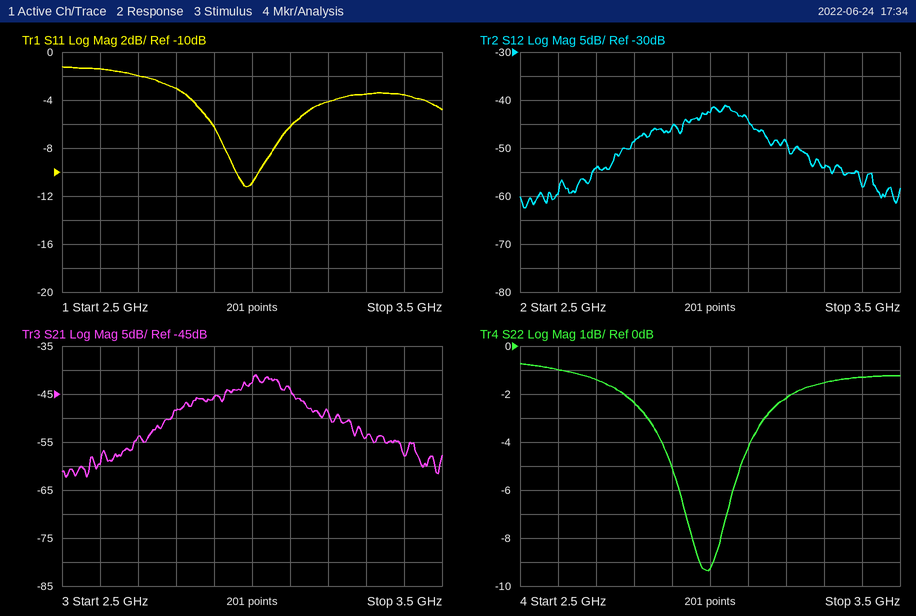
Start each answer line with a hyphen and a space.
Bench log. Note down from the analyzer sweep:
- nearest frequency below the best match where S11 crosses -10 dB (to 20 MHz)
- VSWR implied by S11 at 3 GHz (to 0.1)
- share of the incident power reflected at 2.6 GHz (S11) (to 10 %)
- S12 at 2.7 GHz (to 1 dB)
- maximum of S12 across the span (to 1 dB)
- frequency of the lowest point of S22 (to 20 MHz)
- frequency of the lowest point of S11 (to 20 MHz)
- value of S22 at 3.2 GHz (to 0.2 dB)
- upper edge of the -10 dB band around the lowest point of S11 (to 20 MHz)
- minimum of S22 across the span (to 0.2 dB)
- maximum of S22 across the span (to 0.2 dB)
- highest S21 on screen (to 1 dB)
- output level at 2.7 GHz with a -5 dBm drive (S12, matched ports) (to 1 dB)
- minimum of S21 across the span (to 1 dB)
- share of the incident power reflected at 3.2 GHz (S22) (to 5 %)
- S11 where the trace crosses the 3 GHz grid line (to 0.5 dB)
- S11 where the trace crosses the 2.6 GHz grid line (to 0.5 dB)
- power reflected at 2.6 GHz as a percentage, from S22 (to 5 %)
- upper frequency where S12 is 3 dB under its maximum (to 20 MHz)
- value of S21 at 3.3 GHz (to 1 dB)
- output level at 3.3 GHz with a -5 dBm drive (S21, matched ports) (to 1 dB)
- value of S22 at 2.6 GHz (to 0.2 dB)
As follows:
- 2.96 GHz
- 1.8
- 70 %
- -54 dB
- -41 dB
- 3.00 GHz
- 2.98 GHz
- -2.2 dB
- 3.02 GHz
- -9.4 dB
- -0.8 dB
- -41 dB
- -59 dBm
- -62 dB
- 60 %
- -11.0 dB
- -1.5 dB
- 80 %
- 3.10 GHz
- -54 dB
- -59 dBm
- -1.0 dB
